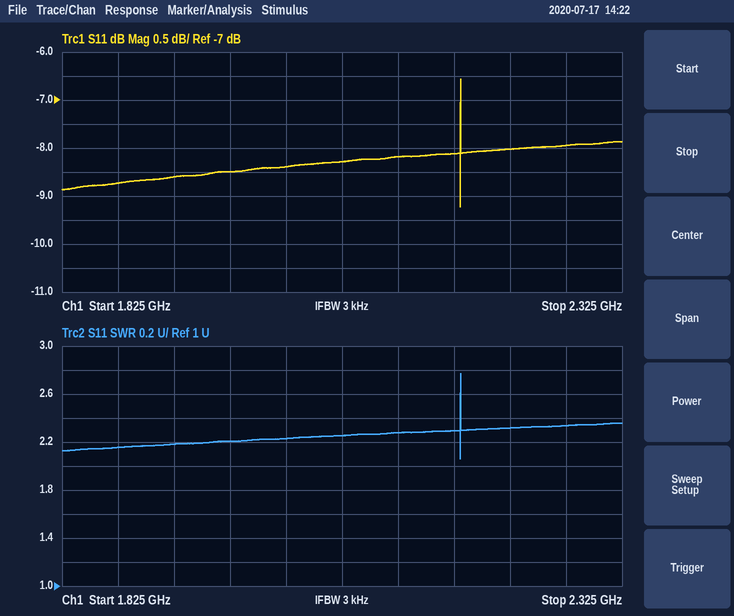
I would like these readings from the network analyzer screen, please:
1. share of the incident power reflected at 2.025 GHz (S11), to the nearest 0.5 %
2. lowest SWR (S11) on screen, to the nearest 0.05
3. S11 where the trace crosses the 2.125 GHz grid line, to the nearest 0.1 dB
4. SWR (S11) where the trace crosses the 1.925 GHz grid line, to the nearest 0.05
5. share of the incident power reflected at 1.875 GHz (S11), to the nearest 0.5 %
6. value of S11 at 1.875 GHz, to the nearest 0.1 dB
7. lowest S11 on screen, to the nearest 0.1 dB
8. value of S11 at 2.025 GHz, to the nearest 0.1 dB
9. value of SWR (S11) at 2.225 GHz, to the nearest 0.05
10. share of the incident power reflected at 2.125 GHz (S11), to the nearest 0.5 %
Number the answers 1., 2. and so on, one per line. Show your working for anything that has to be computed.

1. 10^(-8.4/10) ≈ 14.5 %
2. 2.05
3. -8.2 dB
4. 2.20
5. 10^(-8.7/10) ≈ 13.5 %
6. -8.7 dB
7. -9.2 dB
8. -8.4 dB
9. 2.30
10. 10^(-8.2/10) ≈ 15.1 %, so 15.0 % to the nearest 0.5 %
